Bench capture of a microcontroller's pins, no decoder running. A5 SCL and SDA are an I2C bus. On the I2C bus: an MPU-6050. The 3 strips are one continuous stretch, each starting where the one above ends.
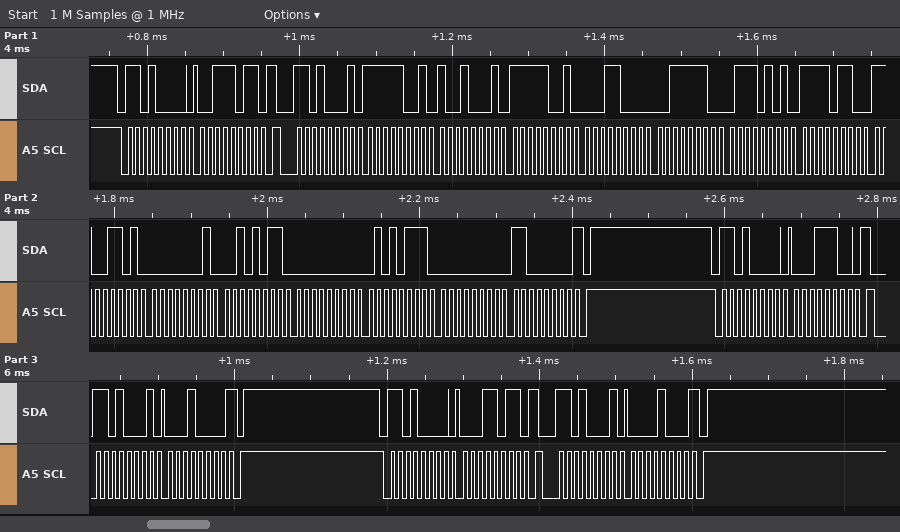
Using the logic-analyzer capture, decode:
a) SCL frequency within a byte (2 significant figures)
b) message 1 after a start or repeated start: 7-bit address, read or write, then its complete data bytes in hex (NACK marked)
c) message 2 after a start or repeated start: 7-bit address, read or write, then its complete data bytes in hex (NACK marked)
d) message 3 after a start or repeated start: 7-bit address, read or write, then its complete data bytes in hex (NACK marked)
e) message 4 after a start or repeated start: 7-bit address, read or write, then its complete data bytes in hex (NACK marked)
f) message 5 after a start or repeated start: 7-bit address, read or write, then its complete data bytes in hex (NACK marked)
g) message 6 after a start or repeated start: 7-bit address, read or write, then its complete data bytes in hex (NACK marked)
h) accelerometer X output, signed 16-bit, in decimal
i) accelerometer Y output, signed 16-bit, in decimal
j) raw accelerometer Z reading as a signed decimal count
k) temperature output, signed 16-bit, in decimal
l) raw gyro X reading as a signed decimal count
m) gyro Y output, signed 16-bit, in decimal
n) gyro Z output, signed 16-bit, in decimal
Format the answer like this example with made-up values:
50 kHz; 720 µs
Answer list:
100 kHz; 0x68 write: 3B; 0x68 read: F9 91 F9 18 3E 75 F6 CD 01 2B 00 57 00 C0 NACK; 0x68 write: 1C; 0x68 read: 10 NACK; 0x68 write: 1B; 0x68 read: 08 NACK; -1647; -1768; 15989; -2355; 299; 87; 192
